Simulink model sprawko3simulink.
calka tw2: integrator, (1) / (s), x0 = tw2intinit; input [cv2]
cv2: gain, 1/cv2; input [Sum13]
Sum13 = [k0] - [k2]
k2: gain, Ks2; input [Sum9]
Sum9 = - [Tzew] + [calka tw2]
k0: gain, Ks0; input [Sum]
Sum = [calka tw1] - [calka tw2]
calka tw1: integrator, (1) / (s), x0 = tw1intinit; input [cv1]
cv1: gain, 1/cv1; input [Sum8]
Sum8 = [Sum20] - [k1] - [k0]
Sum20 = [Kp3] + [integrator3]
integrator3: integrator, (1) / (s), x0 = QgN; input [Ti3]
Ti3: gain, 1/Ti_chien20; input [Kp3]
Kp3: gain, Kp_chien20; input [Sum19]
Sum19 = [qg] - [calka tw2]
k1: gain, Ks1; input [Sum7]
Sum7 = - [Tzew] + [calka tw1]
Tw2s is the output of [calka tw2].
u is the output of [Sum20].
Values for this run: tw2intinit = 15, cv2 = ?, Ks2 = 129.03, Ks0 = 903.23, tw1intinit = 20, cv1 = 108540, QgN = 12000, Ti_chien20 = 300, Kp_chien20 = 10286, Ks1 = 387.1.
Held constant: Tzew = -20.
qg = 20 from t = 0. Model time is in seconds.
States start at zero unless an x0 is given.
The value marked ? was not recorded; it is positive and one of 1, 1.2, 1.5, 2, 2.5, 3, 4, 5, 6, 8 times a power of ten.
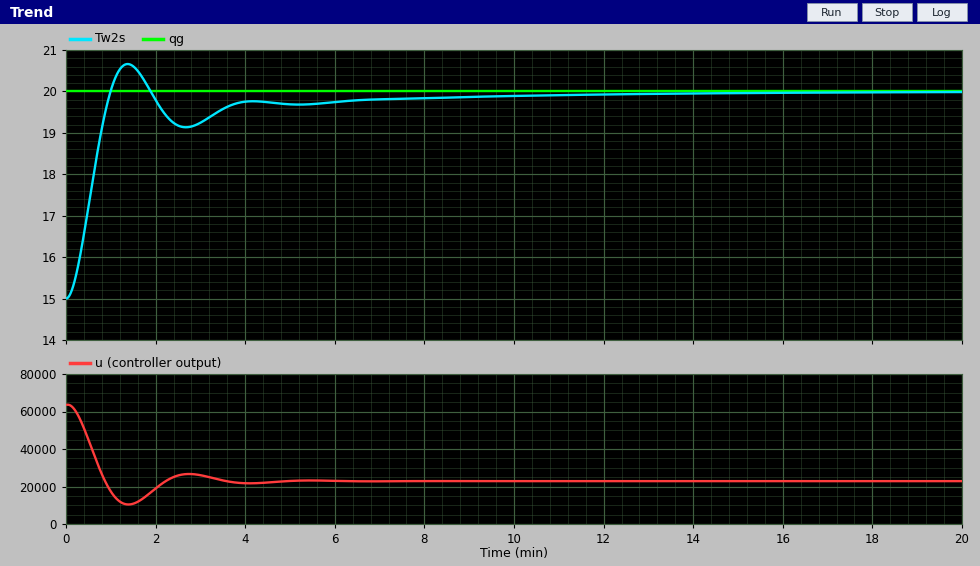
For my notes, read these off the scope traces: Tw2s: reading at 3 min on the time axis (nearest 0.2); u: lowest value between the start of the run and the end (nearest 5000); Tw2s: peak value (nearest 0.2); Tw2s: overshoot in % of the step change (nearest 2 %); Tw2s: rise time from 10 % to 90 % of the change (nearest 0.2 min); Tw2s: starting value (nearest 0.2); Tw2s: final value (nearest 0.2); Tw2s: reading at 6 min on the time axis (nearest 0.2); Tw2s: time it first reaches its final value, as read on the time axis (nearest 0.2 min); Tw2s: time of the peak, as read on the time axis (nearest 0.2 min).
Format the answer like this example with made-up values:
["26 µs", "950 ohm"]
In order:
["19.2", "10000", "20.6", "14 %", "0.6 min", "15.0", "20.0", "19.8", "1.0 min", "1.4 min"]
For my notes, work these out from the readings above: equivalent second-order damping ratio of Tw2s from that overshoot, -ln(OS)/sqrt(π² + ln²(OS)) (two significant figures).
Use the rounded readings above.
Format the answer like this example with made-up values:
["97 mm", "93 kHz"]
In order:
["0.53"]
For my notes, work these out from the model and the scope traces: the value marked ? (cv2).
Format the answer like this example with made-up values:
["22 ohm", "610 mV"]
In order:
["50000"]
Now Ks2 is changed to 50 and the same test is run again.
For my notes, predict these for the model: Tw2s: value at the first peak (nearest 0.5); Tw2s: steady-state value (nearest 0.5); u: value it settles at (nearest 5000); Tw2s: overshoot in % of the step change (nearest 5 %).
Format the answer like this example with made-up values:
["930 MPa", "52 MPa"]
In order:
["21.0", "20.0", "20000", "25 %"]
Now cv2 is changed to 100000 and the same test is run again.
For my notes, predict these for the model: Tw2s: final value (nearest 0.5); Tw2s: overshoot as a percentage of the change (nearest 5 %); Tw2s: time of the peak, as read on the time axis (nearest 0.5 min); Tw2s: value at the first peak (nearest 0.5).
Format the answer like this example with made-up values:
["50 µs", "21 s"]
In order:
["20.0", "20 %", "2.0 min", "21.0"]
